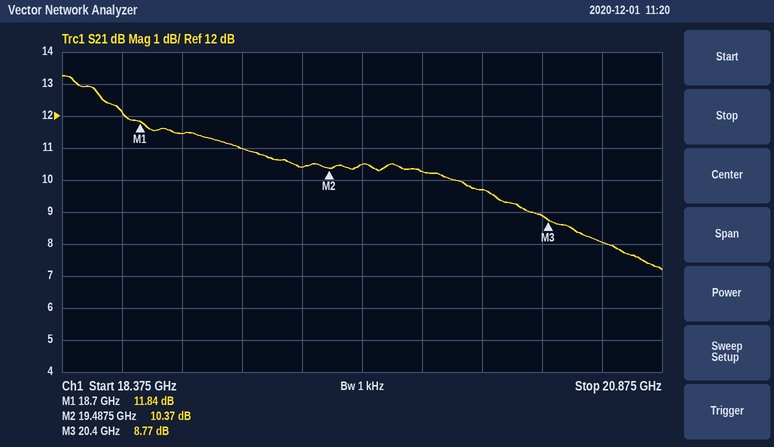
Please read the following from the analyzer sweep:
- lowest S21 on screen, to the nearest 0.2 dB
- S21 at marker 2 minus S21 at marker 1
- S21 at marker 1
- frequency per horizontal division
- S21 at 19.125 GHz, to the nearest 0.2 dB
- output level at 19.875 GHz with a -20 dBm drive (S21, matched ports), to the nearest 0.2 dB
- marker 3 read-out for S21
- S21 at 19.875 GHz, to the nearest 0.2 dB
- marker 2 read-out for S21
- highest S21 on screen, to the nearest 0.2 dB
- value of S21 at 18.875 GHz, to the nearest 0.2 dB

7.2 dB
-1.47 dB
11.84 dB
250 MHz
11.0 dB
-9.8 dBm
8.77 dB
10.2 dB
10.37 dB
13.2 dB
11.4 dB
